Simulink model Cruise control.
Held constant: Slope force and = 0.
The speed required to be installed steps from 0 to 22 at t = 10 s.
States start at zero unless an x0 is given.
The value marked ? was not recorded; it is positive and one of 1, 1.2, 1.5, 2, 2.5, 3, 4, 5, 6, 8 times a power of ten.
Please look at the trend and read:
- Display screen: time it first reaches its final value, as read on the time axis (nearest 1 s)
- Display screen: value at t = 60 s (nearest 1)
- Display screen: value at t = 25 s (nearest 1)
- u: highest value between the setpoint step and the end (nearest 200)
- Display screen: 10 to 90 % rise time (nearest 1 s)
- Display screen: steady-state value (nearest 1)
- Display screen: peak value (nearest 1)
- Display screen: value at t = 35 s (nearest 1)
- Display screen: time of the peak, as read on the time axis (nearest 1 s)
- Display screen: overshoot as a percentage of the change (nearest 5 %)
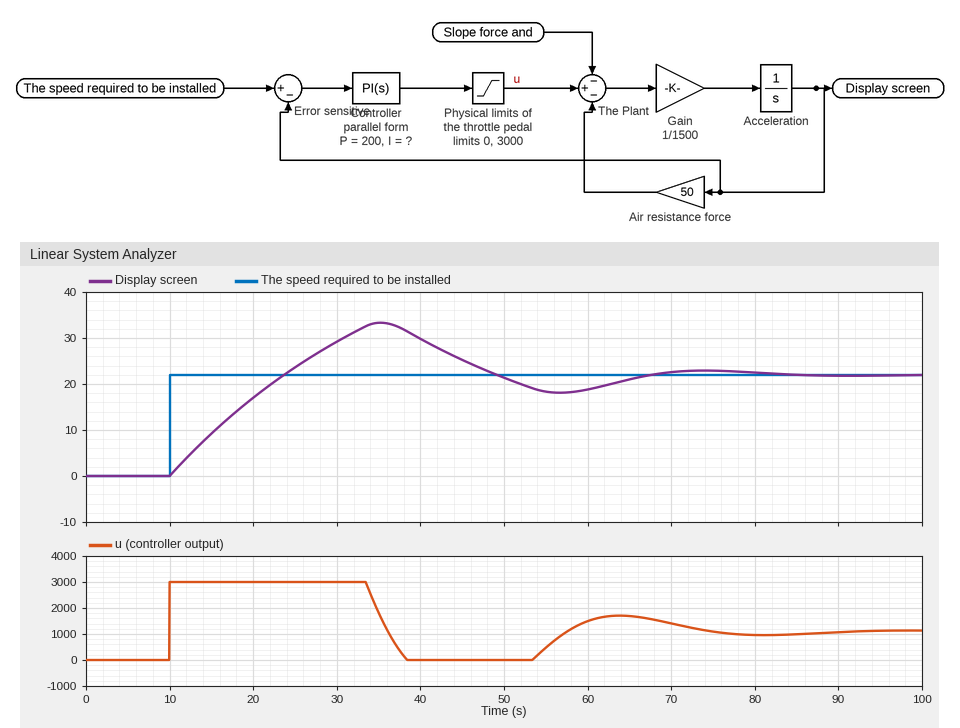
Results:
24 s
19
24
3000
11 s
22
33
33
35 s
50 %
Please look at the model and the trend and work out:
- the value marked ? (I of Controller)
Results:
60
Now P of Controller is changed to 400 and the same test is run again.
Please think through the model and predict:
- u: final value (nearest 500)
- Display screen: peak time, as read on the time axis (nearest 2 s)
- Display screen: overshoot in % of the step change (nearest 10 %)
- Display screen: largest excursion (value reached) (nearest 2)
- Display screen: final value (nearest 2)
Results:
1000
34 s
40 %
32
22
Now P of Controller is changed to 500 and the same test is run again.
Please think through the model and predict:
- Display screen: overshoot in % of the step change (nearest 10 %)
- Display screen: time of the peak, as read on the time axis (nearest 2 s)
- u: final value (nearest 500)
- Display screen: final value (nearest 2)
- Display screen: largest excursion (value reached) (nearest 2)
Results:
40 %
32 s
1000
22
30
